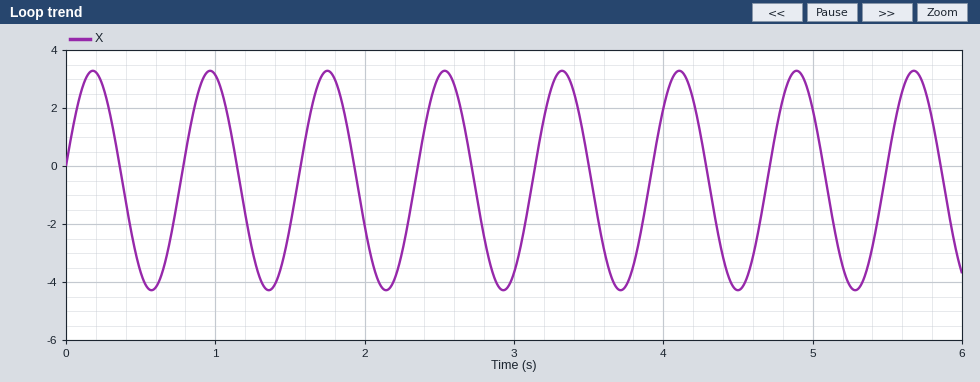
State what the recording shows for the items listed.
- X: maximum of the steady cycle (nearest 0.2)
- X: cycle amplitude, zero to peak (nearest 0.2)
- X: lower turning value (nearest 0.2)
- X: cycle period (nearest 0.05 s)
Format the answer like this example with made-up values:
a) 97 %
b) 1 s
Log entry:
a) 3.2
b) 3.8
c) -4.2
d) 0.80 s
